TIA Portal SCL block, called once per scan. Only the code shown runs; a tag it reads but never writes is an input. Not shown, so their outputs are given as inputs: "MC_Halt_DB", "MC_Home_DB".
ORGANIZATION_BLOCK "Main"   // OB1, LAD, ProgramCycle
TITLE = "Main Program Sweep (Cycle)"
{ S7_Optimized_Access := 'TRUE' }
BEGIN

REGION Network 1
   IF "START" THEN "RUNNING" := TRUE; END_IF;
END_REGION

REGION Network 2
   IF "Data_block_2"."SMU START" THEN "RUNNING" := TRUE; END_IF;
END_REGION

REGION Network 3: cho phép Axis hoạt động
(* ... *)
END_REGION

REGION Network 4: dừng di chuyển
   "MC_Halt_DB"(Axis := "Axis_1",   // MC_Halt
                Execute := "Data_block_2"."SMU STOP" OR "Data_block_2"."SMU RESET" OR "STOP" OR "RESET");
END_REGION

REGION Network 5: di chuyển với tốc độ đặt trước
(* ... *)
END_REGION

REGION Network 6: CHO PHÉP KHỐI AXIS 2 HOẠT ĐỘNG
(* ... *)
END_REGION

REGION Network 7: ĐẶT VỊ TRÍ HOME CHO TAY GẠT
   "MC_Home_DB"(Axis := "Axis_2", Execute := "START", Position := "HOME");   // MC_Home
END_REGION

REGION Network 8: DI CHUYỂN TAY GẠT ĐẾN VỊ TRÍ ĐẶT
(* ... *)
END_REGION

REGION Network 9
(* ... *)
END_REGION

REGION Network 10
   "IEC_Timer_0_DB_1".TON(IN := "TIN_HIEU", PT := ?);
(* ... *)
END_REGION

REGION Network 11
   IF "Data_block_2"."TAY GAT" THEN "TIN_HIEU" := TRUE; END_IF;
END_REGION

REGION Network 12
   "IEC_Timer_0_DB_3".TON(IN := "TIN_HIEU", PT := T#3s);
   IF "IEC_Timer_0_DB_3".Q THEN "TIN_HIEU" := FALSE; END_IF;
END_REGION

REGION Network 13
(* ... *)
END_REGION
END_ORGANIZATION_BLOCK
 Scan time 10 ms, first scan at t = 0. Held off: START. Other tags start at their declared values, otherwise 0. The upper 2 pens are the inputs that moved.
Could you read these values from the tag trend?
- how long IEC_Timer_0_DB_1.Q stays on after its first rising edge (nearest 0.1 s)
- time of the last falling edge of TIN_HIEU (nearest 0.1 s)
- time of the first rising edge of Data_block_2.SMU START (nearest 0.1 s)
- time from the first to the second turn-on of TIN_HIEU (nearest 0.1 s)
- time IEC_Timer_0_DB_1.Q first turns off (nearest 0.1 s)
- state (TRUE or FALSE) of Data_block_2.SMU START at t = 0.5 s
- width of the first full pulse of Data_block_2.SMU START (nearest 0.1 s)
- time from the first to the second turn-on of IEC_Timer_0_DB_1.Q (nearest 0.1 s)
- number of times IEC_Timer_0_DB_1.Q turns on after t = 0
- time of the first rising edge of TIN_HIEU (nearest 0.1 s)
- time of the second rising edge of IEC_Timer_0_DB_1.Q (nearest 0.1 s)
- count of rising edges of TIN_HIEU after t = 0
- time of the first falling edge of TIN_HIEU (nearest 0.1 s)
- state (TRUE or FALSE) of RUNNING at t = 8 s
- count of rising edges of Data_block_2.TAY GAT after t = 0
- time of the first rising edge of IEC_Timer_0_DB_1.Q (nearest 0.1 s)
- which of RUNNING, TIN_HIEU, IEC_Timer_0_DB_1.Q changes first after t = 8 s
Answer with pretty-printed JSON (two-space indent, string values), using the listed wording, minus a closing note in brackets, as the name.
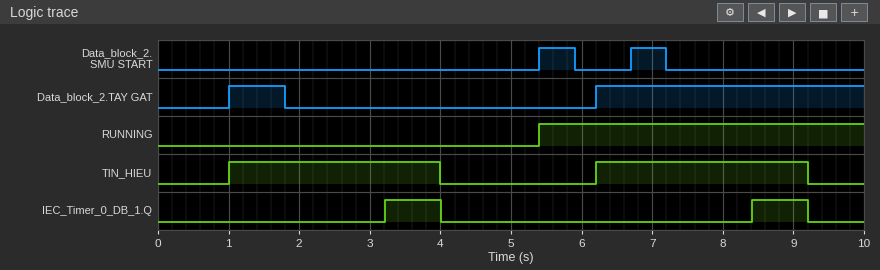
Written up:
{
  "how long IEC_Timer_0_DB_1.Q stays on after its first rising edge": "0.8 s",
  "time of the last falling edge of TIN_HIEU": "9.2 s",
  "time of the first rising edge of Data_block_2.SMU START": "5.4 s",
  "time from the first to the second turn-on of TIN_HIEU": "5.2 s",
  "time IEC_Timer_0_DB_1.Q first turns off": "4.0 s",
  "state (TRUE or FALSE) of Data_block_2.SMU START at t = 0.5 s": "FALSE",
  "width of the first full pulse of Data_block_2.SMU START": "0.5 s",
  "time from the first to the second turn-on of IEC_Timer_0_DB_1.Q": "5.2 s",
  "number of times IEC_Timer_0_DB_1.Q turns on after t = 0": "2",
  "time of the first rising edge of TIN_HIEU": "1.0 s",
  "time of the second rising edge of IEC_Timer_0_DB_1.Q": "8.4 s",
  "count of rising edges of TIN_HIEU after t = 0": "2",
  "time of the first falling edge of TIN_HIEU": "4.0 s",
  "state (TRUE or FALSE) of RUNNING at t = 8 s": "TRUE",
  "count of rising edges of Data_block_2.TAY GAT after t = 0": "2",
  "time of the first rising edge of IEC_Timer_0_DB_1.Q": "3.2 s",
  "which of RUNNING, TIN_HIEU, IEC_Timer_0_DB_1.Q changes first after t = 8 s": "IEC_Timer_0_DB_1.Q"
}
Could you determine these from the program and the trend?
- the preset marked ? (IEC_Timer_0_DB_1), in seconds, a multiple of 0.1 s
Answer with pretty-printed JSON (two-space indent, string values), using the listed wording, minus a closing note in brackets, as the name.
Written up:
{
  "the preset marked ? (IEC_Timer_0_DB_1), in seconds, a multiple of 0.1 s": "2.2 s"
}
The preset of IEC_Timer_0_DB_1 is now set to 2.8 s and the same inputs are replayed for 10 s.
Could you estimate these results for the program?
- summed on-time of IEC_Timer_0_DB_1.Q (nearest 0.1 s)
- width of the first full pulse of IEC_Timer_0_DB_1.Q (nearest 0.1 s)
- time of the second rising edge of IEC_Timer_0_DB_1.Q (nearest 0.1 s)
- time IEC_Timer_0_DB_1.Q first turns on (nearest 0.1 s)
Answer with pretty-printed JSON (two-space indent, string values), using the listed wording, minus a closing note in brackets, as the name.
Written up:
{
  "summed on-time of IEC_Timer_0_DB_1.Q": "0.4 s",
  "width of the first full pulse of IEC_Timer_0_DB_1.Q": "0.2 s",
  "time of the second rising edge of IEC_Timer_0_DB_1.Q": "9.0 s",
  "time IEC_Timer_0_DB_1.Q first turns on": "3.8 s"
}
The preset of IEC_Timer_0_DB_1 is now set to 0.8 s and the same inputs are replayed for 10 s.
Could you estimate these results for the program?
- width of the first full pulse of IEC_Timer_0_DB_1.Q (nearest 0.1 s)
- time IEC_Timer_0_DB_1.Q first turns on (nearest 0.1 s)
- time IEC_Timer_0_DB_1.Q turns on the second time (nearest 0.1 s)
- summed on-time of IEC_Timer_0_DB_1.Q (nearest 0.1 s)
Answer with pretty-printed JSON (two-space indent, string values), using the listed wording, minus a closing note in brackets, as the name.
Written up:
{
  "width of the first full pulse of IEC_Timer_0_DB_1.Q": "2.2 s",
  "time IEC_Timer_0_DB_1.Q first turns on": "1.8 s",
  "time IEC_Timer_0_DB_1.Q turns on the second time": "7.0 s",
  "summed on-time of IEC_Timer_0_DB_1.Q": "4.4 s"
}
